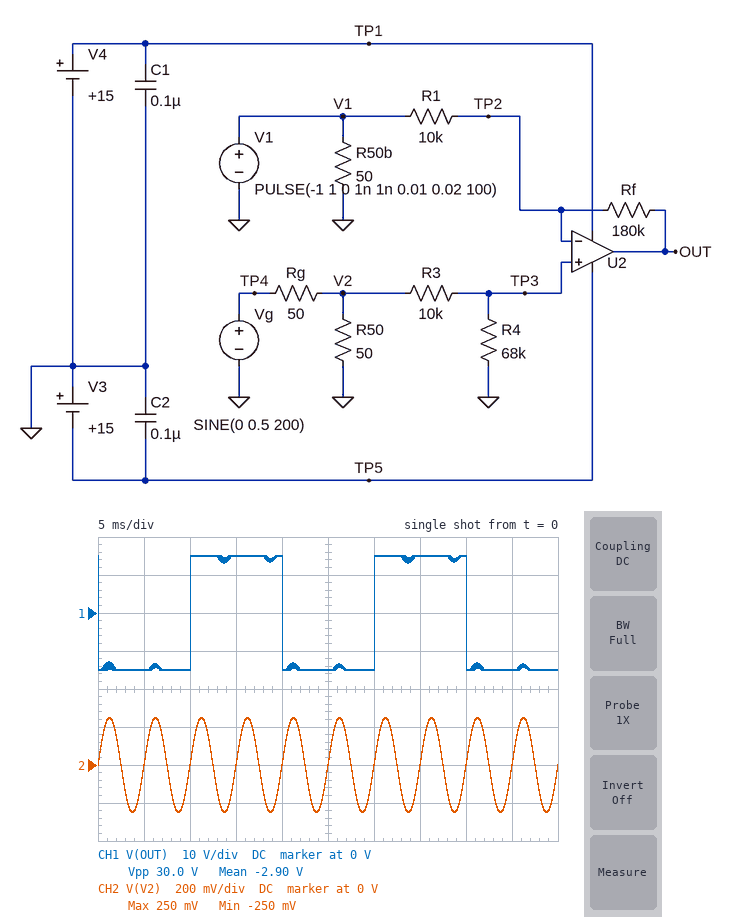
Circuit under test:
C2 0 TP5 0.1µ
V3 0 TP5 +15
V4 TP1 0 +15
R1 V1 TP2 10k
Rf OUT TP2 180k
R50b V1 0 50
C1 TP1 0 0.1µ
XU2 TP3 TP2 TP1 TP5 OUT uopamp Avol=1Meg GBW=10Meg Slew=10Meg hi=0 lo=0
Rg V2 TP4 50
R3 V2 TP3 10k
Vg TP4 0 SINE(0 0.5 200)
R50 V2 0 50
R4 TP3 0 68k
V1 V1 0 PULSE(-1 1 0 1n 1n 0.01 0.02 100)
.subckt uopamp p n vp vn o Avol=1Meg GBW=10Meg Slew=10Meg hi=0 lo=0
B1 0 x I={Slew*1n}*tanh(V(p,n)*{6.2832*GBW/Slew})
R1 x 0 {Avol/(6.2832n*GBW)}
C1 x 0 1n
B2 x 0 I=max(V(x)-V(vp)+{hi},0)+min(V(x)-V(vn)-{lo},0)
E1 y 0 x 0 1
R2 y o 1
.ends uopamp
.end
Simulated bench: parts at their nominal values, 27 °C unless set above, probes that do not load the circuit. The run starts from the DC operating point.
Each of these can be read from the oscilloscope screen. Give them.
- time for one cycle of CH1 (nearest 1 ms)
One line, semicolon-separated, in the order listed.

20 ms
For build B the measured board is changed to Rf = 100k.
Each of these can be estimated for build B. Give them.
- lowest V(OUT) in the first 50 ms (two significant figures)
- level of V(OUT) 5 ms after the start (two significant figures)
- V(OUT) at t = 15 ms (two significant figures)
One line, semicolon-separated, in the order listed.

-12 V; -10 V; 10 V
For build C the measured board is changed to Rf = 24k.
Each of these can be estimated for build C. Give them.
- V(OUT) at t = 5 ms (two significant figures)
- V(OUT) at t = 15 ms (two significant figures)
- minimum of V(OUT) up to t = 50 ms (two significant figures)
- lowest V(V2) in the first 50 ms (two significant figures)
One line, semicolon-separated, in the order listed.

-2.4 V; 2.4 V; -3.1 V; -250 mV
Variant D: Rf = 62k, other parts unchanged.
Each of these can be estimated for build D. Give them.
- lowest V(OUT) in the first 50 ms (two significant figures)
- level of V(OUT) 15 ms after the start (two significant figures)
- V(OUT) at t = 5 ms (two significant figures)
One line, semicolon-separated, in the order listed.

-7.8 V; 6.2 V; -6.2 V
